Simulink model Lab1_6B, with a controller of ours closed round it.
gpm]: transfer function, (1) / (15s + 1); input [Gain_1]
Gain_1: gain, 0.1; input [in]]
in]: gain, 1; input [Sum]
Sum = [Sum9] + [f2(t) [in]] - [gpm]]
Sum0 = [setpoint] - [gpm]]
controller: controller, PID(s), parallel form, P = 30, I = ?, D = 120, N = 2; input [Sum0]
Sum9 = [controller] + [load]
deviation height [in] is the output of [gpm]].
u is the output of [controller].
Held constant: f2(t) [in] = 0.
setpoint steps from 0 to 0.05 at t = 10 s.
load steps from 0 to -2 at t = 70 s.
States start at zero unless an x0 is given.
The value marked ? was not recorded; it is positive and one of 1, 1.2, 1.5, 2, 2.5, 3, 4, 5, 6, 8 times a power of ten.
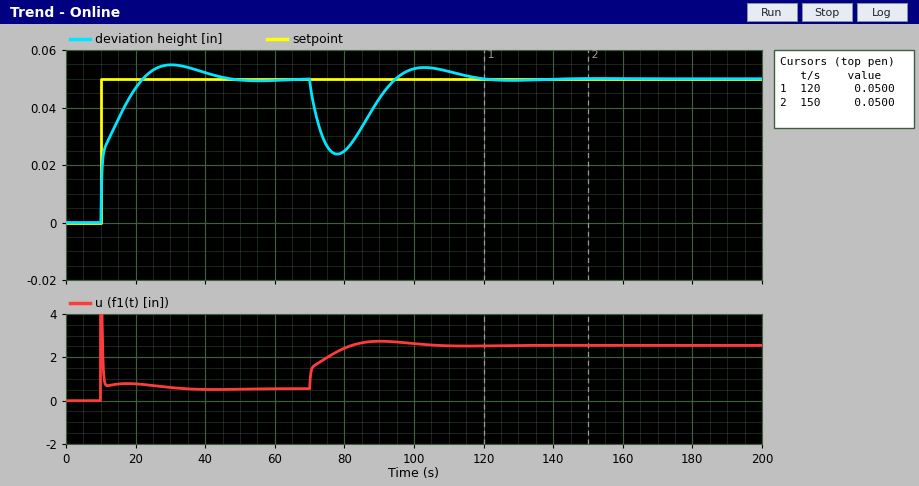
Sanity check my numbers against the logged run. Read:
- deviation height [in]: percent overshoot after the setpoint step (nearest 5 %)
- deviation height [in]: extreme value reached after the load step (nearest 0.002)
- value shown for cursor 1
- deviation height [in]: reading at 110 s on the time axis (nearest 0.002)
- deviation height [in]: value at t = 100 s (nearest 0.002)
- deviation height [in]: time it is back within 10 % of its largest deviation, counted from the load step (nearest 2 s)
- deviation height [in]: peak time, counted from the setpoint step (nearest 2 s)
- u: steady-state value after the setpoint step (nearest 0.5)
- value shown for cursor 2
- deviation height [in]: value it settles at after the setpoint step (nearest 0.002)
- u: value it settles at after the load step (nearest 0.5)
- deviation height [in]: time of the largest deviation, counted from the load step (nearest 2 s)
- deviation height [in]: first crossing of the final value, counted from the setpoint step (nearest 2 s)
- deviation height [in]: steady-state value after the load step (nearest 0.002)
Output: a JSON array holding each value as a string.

["10 %", "0.024", "0.0500", "0.052", "0.054", "40 s", "20 s", "0.5", "0.0500", "0.050", "2.5", "8 s", "12 s", "0.050"]
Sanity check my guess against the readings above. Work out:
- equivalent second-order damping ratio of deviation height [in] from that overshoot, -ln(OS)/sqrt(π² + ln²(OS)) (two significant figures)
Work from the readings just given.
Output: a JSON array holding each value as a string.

["0.59"]
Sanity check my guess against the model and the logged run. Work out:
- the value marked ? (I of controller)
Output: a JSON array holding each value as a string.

["6"]
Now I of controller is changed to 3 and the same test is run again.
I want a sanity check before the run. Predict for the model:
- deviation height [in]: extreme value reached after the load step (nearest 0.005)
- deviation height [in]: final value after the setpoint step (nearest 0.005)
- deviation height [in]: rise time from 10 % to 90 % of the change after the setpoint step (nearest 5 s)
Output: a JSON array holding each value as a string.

["0.020", "0.050", "15 s"]
